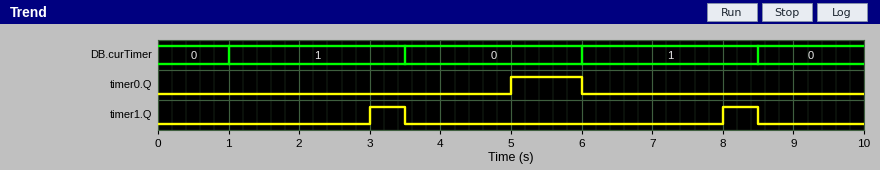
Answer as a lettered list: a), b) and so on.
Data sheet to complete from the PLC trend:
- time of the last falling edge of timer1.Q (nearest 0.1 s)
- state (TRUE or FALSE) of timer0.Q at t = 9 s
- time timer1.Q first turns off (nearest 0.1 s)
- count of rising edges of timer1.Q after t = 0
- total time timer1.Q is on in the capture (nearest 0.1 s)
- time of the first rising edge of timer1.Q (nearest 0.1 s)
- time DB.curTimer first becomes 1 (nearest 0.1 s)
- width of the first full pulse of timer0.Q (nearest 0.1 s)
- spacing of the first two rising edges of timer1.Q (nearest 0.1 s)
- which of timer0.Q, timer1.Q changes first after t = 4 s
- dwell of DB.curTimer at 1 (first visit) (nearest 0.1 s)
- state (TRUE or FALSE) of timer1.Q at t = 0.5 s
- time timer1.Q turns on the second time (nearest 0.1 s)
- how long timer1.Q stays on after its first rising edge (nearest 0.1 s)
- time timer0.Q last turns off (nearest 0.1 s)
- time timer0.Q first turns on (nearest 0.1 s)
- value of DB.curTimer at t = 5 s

a) 8.5 s
b) FALSE
c) 3.5 s
d) 2
e) 1.0 s
f) 3.0 s
g) 1.0 s
h) 1.0 s
i) 5.0 s
j) timer0.Q
k) 2.5 s
l) FALSE
m) 8.0 s
n) 0.5 s
o) 6.0 s
p) 5.0 s
q) 0
